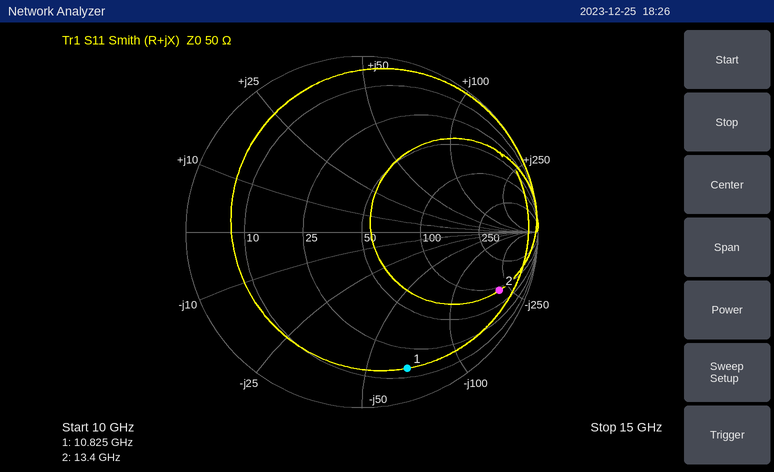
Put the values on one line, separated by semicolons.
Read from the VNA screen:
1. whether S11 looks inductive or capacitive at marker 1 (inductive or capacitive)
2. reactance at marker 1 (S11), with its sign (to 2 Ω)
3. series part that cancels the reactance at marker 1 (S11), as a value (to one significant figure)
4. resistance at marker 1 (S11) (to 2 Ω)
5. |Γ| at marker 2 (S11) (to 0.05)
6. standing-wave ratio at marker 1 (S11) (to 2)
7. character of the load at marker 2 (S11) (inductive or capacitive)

capacitive; -68 Ω; 1.0 nH; 14 Ω; 0.85; 10; capacitive
